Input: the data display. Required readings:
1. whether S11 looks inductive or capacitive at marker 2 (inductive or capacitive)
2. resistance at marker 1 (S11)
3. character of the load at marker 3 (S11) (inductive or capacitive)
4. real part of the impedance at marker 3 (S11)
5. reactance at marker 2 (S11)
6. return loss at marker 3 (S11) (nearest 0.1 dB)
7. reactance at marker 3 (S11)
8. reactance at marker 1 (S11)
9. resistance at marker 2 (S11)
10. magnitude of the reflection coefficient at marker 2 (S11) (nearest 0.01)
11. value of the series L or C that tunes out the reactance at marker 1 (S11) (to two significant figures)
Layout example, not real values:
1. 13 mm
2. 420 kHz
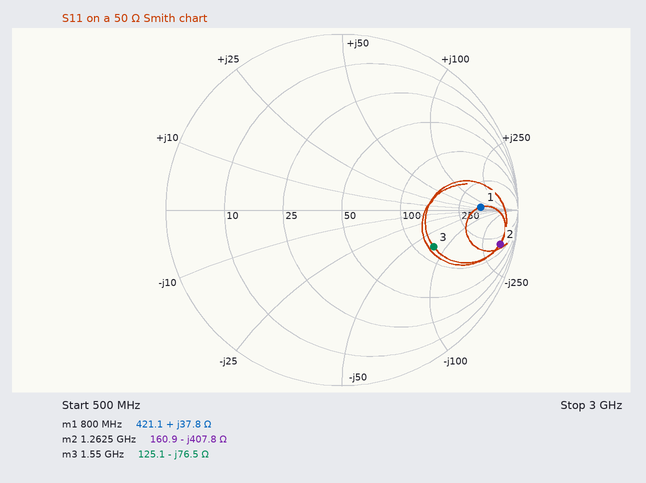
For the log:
1. capacitive
2. 421.1 Ω
3. capacitive
4. 125.1 Ω
5. -407.8 Ω
6. 5.0 dB
7. -76.5 Ω
8. +37.8 Ω
9. 160.9 Ω
10. 0.92
11. 5.3 pF
